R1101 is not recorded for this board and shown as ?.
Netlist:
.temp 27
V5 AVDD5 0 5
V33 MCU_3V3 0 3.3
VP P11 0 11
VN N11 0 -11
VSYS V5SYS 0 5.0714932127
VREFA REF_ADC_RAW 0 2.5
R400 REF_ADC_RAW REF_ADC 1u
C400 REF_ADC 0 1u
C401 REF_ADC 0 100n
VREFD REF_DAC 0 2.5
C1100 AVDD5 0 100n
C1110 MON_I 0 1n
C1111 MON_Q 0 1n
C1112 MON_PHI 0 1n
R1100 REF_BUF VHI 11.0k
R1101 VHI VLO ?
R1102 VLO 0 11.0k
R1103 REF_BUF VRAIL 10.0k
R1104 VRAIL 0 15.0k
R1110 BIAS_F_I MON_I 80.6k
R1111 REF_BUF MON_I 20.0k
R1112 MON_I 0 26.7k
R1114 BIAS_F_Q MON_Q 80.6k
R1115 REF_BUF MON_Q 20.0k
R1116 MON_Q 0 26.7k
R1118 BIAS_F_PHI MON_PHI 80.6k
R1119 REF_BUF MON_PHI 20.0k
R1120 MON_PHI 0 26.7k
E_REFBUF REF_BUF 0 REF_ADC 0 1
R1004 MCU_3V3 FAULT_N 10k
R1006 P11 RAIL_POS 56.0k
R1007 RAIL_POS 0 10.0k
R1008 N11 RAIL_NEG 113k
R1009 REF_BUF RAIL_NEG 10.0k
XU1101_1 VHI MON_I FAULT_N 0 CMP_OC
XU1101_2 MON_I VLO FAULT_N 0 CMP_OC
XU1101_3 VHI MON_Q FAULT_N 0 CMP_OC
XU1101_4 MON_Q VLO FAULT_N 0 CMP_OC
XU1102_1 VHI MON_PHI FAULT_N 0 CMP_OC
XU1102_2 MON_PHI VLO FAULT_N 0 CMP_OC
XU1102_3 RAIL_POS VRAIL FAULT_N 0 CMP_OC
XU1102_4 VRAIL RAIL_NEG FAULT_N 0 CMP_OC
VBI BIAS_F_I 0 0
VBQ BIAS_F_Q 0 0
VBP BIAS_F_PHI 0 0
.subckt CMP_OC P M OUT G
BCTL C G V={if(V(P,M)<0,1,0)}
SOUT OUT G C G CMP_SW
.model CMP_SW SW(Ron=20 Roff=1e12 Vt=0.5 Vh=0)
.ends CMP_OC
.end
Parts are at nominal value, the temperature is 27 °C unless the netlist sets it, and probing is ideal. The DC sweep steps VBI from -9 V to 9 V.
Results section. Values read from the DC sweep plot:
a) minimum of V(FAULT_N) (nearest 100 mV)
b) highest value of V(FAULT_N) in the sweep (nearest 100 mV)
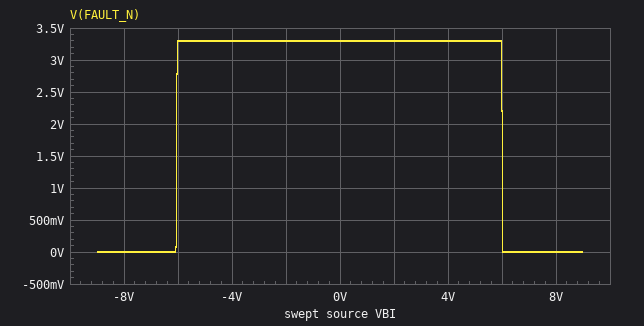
0 V
3.3 V
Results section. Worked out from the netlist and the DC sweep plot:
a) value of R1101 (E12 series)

33 kΩ
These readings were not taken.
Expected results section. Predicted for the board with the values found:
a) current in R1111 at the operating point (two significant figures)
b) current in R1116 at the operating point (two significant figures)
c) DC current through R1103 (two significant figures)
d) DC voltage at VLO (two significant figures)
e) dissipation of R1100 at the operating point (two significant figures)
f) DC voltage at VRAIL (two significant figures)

62 µA
47 µA
100 µA
500 mV
23 µW
1.5 V
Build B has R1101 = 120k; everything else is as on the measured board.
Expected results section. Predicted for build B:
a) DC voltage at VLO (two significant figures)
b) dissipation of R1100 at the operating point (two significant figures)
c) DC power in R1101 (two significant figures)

190 mV
3.4 µW
37 µW
